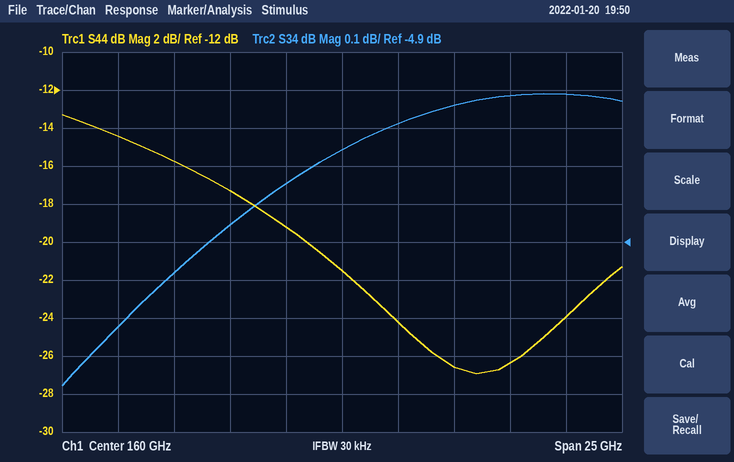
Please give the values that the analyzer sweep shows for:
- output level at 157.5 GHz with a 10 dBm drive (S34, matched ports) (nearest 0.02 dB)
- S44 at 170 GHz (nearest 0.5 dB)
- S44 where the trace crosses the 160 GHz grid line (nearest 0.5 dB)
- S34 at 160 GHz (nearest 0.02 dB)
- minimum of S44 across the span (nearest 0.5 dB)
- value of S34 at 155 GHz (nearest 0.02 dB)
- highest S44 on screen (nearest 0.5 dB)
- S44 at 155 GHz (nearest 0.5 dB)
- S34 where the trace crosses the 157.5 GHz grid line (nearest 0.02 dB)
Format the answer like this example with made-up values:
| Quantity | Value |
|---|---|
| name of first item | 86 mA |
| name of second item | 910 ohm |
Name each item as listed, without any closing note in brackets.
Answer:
| Quantity | Value |
|---|---|
| output level at 157.5 GHz with a 10 dBm drive (S34, matched ports) | 5.26 dBm |
| S44 at 170 GHz | -24.0 dB |
| S44 where the trace crosses the 160 GHz grid line | -21.5 dB |
| S34 at 160 GHz | -4.66 dB |
| minimum of S44 across the span | -27.0 dB |
| value of S34 at 155 GHz | -4.86 dB |
| highest S44 on screen | -13.5 dB |
| S44 at 155 GHz | -17.5 dB |
| S34 where the trace crosses the 157.5 GHz grid line | -4.74 dB |
